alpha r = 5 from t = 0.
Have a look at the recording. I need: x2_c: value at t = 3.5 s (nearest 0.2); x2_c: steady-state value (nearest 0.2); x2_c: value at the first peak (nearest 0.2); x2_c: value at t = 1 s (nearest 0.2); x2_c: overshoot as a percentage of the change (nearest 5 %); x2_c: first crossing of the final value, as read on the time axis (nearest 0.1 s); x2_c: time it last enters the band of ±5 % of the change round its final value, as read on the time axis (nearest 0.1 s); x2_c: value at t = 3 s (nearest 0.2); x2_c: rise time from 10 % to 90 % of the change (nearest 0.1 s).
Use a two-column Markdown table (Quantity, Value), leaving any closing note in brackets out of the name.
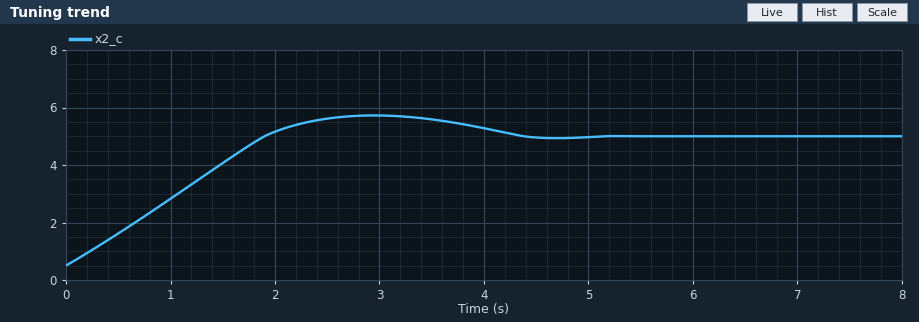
| Quantity | Value |
|---|---|
| x2_c: value at t = 3.5 s | 5.6 |
| x2_c: steady-state value | 5.0 |
| x2_c: value at the first peak | 5.8 |
| x2_c: value at t = 1 s | 2.8 |
| x2_c: overshoot as a percentage of the change | 15 % |
| x2_c: first crossing of the final value, as read on the time axis | 1.9 s |
| x2_c: time it last enters the band of ±5 % of the change round its final value, as read on the time axis | 4.1 s |
| x2_c: value at t = 3 s | 5.8 |
| x2_c: rise time from 10 % to 90 % of the change | 1.5 s |
